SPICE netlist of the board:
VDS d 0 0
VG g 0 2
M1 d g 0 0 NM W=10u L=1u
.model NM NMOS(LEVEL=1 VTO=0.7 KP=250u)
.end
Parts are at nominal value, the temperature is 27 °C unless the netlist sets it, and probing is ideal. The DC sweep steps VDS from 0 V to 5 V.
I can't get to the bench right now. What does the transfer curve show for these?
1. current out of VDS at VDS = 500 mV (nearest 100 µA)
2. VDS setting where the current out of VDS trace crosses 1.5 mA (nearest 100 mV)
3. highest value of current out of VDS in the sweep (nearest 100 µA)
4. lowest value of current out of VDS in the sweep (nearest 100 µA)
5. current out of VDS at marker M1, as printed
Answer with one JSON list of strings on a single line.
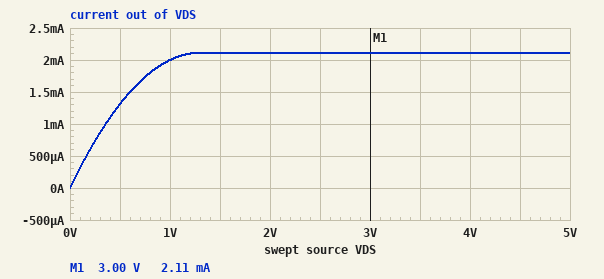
["1.3 mA", "600 mV", "2.1 mA", "0 A", "2.11 mA"]
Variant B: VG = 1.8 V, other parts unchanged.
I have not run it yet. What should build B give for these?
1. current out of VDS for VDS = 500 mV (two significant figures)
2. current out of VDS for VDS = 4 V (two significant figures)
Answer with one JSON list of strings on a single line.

["1.1 mA", "1.5 mA"]
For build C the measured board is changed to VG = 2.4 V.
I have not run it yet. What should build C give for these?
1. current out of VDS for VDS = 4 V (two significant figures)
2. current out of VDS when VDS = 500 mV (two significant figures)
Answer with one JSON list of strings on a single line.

["3.6 mA", "1.8 mA"]
